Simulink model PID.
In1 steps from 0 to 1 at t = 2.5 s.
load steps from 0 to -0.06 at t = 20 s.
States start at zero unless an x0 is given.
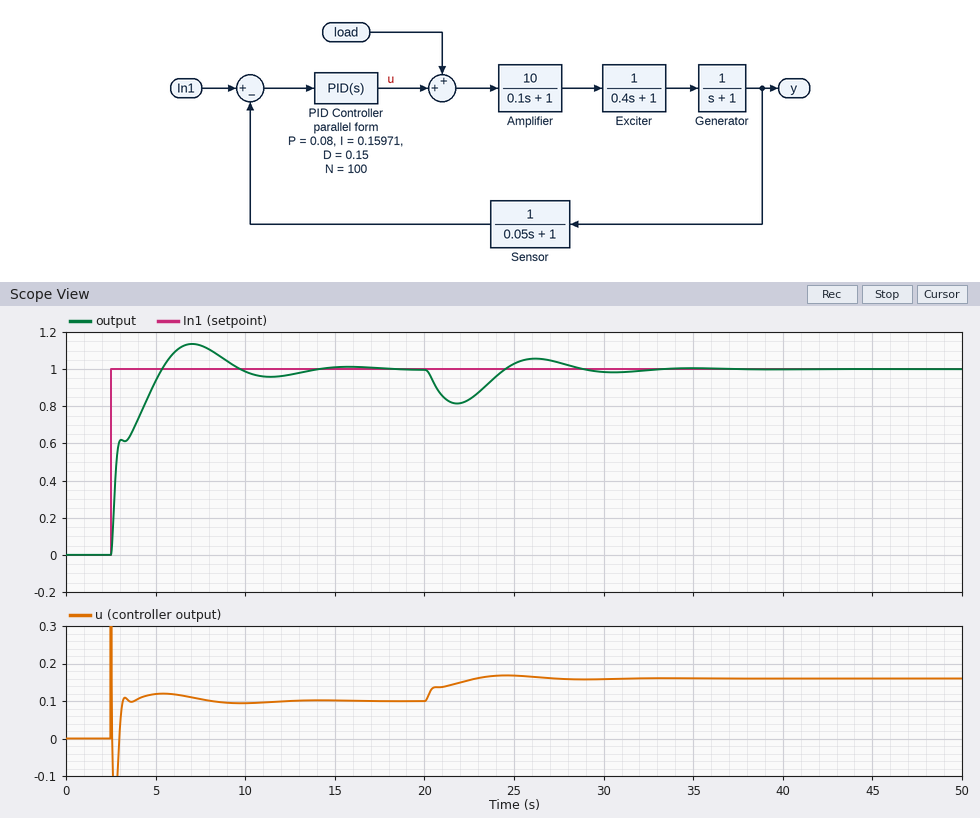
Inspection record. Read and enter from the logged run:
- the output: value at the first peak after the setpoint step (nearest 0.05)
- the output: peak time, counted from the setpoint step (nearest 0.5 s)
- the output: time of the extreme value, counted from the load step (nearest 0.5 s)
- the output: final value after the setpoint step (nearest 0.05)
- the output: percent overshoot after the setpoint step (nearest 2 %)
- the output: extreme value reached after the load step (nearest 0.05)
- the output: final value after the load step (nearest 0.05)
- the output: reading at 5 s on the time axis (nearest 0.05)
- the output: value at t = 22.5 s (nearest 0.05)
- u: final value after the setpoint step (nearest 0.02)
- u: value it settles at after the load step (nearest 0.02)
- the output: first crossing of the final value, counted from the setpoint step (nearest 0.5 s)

1.15
4.5 s
2.0 s
1.00
14 %
0.80
1.00
0.95
0.85
0.10
0.16
3.0 s
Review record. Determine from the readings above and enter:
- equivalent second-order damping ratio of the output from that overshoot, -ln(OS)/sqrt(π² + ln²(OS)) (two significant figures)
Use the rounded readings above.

0.53
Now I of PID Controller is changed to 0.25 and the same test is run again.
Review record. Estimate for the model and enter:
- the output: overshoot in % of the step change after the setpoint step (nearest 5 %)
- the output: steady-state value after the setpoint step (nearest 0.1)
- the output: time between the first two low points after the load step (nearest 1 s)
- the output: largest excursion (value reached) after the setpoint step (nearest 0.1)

20 %
1.0
7 s
1.2
